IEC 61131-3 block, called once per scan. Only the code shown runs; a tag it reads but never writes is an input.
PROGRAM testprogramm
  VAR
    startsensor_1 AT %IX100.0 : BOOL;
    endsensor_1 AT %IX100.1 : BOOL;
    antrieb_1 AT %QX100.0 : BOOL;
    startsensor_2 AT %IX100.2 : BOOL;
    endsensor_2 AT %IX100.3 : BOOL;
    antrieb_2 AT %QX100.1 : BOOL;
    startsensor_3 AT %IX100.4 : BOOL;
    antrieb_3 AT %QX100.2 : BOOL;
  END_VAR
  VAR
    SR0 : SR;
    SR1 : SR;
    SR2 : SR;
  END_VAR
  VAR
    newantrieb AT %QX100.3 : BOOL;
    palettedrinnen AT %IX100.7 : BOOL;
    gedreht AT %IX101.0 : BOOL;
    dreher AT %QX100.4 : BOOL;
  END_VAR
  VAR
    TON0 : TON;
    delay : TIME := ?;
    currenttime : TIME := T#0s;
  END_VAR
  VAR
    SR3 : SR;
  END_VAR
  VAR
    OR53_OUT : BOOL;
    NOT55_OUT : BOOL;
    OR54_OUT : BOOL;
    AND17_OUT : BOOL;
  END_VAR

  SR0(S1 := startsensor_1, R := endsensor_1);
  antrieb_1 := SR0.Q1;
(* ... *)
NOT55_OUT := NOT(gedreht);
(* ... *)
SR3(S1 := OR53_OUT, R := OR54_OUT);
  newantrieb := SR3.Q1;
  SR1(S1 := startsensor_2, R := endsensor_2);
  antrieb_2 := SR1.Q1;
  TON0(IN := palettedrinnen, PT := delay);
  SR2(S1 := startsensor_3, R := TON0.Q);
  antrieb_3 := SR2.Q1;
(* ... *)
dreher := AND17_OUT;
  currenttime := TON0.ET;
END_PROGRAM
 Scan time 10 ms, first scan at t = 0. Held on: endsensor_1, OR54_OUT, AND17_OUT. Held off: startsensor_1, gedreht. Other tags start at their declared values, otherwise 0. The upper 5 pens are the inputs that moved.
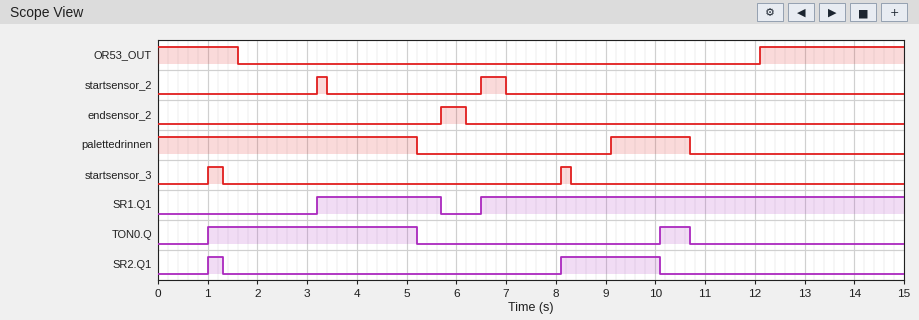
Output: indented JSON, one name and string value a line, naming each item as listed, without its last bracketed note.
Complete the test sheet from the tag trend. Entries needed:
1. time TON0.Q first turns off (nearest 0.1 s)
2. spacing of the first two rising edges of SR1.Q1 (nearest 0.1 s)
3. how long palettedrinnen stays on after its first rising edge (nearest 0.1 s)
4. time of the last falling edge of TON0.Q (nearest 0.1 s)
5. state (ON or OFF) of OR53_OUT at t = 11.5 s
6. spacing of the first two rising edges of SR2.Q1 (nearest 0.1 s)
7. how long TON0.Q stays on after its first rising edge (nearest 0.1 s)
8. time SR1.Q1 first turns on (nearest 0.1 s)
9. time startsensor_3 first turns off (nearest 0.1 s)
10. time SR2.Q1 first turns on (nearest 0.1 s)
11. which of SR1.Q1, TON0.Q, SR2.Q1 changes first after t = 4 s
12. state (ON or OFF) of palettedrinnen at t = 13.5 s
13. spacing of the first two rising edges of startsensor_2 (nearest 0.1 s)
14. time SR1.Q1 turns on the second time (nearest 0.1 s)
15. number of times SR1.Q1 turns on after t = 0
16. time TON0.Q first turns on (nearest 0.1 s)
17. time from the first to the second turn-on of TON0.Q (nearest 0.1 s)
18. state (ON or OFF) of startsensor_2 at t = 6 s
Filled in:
{
  "time TON0.Q first turns off": "5.2 s",
  "spacing of the first two rising edges of SR1.Q1": "3.3 s",
  "how long palettedrinnen stays on after its first rising edge": "1.6 s",
  "time of the last falling edge of TON0.Q": "10.7 s",
  "state (ON or OFF) of OR53_OUT at t = 11.5 s": "OFF",
  "spacing of the first two rising edges of SR2.Q1": "7.1 s",
  "how long TON0.Q stays on after its first rising edge": "4.2 s",
  "time SR1.Q1 first turns on": "3.2 s",
  "time startsensor_3 first turns off": "1.3 s",
  "time SR2.Q1 first turns on": "1.0 s",
  "which of SR1.Q1, TON0.Q, SR2.Q1 changes first after t = 4 s": "TON0.Q",
  "state (ON or OFF) of palettedrinnen at t = 13.5 s": "OFF",
  "spacing of the first two rising edges of startsensor_2": "3.3 s",
  "time SR1.Q1 turns on the second time": "6.5 s",
  "number of times SR1.Q1 turns on after t = 0": "2",
  "time TON0.Q first turns on": "1.0 s",
  "time from the first to the second turn-on of TON0.Q": "9.1 s",
  "state (ON or OFF) of startsensor_2 at t = 6 s": "OFF"
}
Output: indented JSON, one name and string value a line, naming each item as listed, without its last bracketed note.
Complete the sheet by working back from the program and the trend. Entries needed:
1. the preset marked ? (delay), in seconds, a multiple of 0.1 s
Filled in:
{
  "the preset marked ? (delay), in seconds, a multiple of 0.1 s": "1.0 s"
}
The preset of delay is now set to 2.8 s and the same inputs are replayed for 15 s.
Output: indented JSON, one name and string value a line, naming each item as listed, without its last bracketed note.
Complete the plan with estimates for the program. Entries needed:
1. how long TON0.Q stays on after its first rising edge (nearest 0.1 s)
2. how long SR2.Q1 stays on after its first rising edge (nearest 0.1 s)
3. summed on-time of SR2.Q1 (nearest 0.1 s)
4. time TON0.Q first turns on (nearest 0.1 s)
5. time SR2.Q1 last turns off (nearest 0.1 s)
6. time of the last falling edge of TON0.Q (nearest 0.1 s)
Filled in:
{
  "how long TON0.Q stays on after its first rising edge": "2.4 s",
  "how long SR2.Q1 stays on after its first rising edge": "1.8 s",
  "summed on-time of SR2.Q1": "8.7 s",
  "time TON0.Q first turns on": "2.8 s",
  "time SR2.Q1 last turns off": "2.8 s",
  "time of the last falling edge of TON0.Q": "5.2 s"
}
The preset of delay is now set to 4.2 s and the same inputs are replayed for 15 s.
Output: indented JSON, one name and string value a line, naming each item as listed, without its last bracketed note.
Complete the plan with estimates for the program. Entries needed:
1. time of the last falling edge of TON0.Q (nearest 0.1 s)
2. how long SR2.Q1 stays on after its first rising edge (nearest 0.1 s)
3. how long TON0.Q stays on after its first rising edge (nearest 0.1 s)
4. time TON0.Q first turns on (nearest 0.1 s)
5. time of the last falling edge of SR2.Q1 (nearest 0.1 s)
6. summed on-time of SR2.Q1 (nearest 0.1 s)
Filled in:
{
  "time of the last falling edge of TON0.Q": "5.2 s",
  "how long SR2.Q1 stays on after its first rising edge": "3.2 s",
  "how long TON0.Q stays on after its first rising edge": "1.0 s",
  "time TON0.Q first turns on": "4.2 s",
  "time of the last falling edge of SR2.Q1": "4.2 s",
  "summed on-time of SR2.Q1": "10.1 s"
}
